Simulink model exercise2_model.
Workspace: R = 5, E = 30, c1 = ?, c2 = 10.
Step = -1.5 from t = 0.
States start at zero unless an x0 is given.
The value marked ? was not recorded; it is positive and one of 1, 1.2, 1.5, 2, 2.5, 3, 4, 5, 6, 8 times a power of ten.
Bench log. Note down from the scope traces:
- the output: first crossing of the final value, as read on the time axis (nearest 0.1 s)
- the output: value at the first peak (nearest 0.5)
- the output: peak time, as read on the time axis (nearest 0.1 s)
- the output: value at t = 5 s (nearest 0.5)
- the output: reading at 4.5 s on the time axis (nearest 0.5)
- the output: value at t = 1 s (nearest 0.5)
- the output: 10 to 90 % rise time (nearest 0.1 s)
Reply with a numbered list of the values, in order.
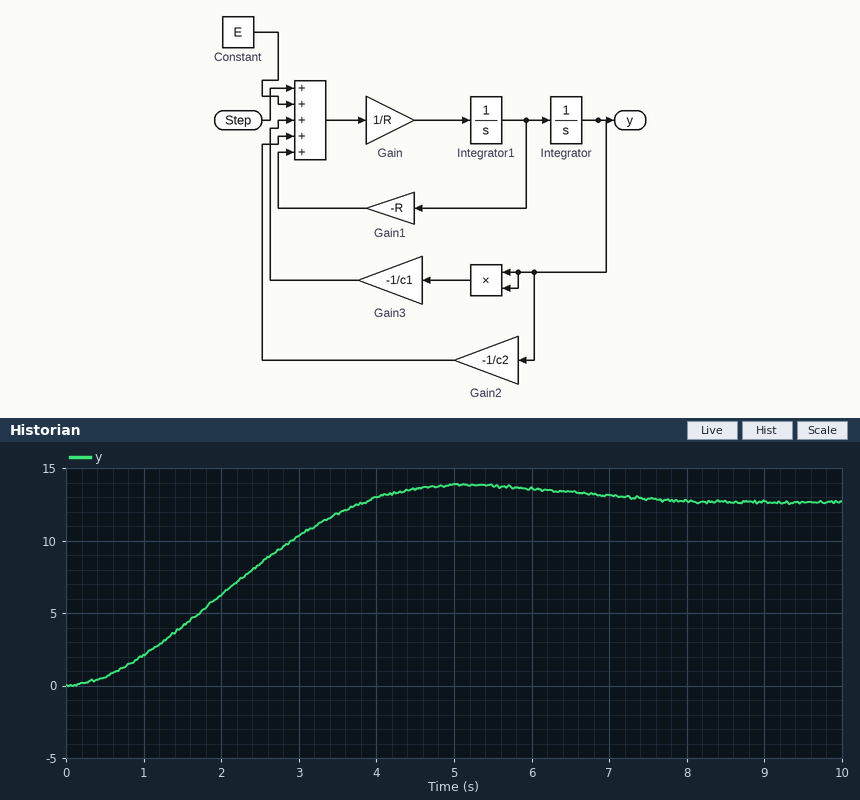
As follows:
1. 3.9 s
2. 14.0
3. 5.2 s
4. 14.0
5. 13.5
6. 2.0
7. 2.6 s
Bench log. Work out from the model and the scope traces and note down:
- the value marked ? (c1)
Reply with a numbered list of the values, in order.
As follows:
1. 6
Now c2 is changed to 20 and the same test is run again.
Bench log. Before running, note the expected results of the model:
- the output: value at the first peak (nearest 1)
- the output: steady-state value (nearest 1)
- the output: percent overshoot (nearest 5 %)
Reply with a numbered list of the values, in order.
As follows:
1. 14
2. 13
3. 10 %
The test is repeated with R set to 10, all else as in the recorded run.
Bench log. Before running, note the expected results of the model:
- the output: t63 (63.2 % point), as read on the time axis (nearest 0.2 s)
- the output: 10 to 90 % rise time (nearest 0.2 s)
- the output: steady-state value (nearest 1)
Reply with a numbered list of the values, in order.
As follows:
1. 4.0 s
2. 5.2 s
3. 13
